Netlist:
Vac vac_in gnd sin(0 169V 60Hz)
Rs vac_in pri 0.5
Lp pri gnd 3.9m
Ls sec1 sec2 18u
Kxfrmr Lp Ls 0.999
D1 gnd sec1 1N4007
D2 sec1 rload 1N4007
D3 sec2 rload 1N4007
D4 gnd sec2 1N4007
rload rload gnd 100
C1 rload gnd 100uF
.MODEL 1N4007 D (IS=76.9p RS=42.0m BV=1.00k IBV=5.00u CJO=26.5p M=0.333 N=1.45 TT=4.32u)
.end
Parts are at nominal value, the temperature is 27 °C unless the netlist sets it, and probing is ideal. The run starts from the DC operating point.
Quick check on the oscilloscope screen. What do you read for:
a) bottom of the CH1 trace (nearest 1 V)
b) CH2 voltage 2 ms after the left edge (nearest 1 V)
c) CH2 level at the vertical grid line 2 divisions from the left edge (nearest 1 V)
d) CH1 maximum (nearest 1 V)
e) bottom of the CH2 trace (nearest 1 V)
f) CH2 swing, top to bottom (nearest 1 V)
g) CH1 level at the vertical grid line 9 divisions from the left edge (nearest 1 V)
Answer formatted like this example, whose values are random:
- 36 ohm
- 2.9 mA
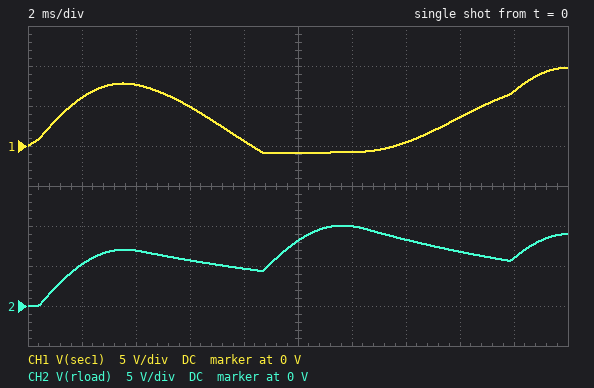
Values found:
- -1 V
- 5 V
- 7 V
- 10 V
- 0 V
- 10 V
- 7 V
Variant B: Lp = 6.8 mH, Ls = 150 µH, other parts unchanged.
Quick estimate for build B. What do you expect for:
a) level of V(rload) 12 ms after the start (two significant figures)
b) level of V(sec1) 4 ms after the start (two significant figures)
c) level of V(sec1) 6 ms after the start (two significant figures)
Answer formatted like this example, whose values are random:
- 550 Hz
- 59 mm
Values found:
- 25 V
- 20 V
- 14 V
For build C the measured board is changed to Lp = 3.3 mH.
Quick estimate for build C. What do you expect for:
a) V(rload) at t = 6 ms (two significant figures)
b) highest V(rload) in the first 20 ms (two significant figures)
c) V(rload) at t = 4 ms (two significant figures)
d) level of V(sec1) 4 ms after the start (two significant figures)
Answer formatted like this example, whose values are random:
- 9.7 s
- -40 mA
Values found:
- 5.9 V
- 11 V
- 7.2 V
- 7.9 V
